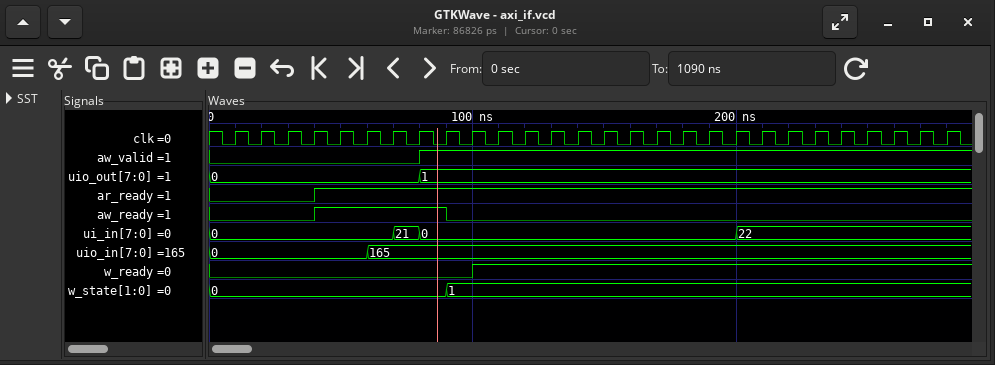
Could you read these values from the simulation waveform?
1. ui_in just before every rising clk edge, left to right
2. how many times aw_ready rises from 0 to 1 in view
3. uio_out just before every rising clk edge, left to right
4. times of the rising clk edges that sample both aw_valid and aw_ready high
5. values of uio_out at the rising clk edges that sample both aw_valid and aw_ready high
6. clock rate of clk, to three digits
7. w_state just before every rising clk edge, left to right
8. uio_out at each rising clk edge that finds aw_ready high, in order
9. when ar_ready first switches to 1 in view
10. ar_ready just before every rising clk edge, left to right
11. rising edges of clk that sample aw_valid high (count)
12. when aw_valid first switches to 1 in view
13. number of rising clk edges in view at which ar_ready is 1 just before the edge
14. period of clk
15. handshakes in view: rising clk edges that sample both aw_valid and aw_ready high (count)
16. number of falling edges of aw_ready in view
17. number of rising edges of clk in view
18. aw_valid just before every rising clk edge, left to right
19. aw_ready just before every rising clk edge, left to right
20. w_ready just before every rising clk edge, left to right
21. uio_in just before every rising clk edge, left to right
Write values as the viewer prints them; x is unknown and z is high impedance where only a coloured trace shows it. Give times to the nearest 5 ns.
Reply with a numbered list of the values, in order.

1. 0, 0, 0, 0, 0, 0, 0, 21, 0, 0, 0, 0, 0, 0, 0, 0, 0, 0, 0, 0, 22, 22, 22, 22, 22, 22, 22, 22
2. 1
3. 0, 0, 0, 0, 0, 0, 0, 0, 1, 1, 1, 1, 1, 1, 1, 1, 1, 1, 1, 1, 1, 1, 1, 1, 1, 1, 1, 1
4. 90 ns
5. 1
6. 100 MHz
7. 0, 0, 0, 0, 0, 0, 0, 0, 0, 1, 1, 1, 1, 1, 1, 1, 1, 1, 1, 1, 1, 1, 1, 1, 1, 1, 1, 1
8. 0, 0, 0, 0, 1
9. 40 ns
10. 0 0 0 0 1 1 1 1 1 1 1 1 1 1 1 1 1 1 1 1 1 1 1 1 1 1 1 1
11. 20
12. 80 ns
13. 24
14. 10 ns
15. 1
16. 1
17. 28
18. 0 0 0 0 0 0 0 0 1 1 1 1 1 1 1 1 1 1 1 1 1 1 1 1 1 1 1 1
19. 0 0 0 0 1 1 1 1 1 0 0 0 0 0 0 0 0 0 0 0 0 0 0 0 0 0 0 0
20. 0 0 0 0 0 0 0 0 0 0 1 1 1 1 1 1 1 1 1 1 1 1 1 1 1 1 1 1
21. 0, 0, 0, 0, 0, 0, 165, 165, 165, 165, 165, 165, 165, 165, 165, 165, 165, 165, 165, 165, 165, 165, 165, 165, 165, 165, 165, 165
